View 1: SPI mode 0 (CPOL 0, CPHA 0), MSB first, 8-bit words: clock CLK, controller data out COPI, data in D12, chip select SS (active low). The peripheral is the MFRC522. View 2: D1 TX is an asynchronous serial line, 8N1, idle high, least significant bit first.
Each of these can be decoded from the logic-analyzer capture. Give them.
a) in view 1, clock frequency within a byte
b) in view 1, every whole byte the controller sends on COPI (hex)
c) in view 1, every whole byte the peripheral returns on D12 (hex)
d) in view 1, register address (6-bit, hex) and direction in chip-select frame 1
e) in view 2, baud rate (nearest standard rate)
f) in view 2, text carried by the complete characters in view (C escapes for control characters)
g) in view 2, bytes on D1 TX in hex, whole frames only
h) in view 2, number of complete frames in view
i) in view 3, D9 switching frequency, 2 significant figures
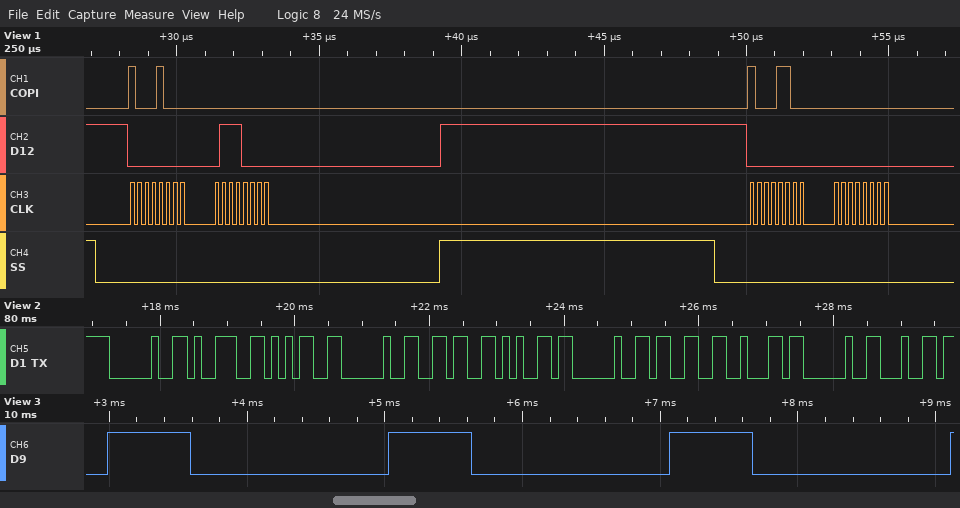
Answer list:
4 MHz
88 00 8C 00
00 70 00 00
0x04 read
9600 baud
" 95 6e 3b d"
0x20 0x39 0x35 0x20 0x36 0x65 0x20 0x33 0x62 0x20 0x64
11
490 Hz
